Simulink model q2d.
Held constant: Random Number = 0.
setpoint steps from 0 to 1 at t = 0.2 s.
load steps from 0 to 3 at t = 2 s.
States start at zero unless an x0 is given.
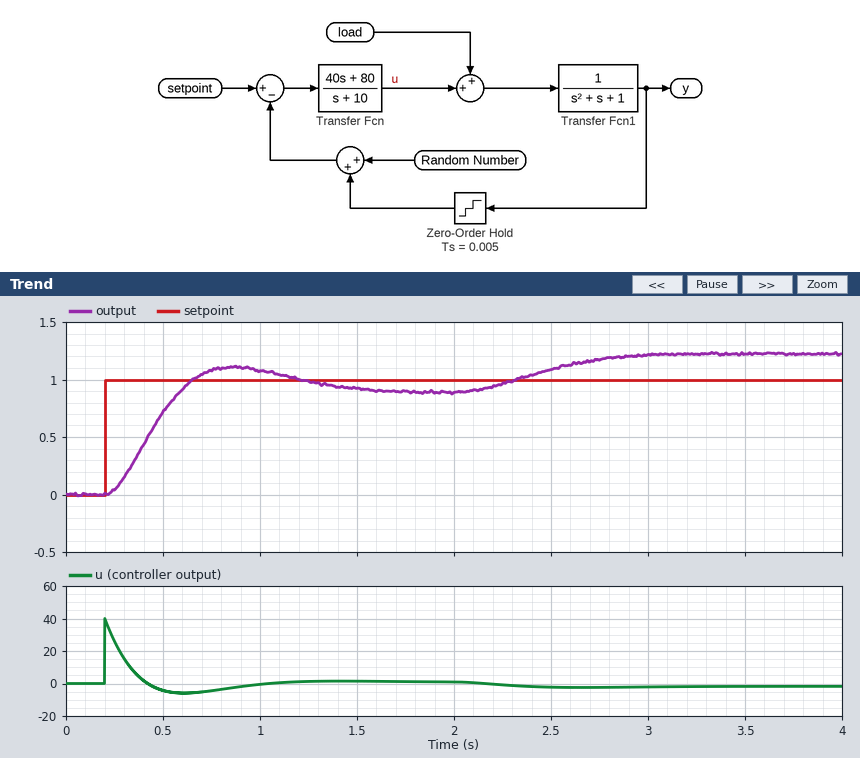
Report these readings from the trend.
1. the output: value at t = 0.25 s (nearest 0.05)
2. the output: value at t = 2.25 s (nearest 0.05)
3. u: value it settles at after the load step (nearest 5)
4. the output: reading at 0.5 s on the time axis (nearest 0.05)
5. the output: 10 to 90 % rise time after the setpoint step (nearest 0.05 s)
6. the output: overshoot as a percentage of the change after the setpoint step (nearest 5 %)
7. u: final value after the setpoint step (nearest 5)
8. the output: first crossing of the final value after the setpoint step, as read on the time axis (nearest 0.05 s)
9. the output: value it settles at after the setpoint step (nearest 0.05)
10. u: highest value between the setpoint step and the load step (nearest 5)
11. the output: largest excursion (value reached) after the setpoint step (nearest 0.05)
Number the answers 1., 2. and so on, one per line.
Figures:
1. 0.05
2. 0.95
3. 0
4. 0.70
5. 0.25 s
6. 25 %
7. 0
8. 0.60 s
9. 0.90
10. 40
11. 1.10
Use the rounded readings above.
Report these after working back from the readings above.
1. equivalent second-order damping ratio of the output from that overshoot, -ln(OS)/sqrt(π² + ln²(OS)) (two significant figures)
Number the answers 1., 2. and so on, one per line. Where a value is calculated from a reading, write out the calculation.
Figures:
1. ln(0.25) = -1.386; 1.386 / sqrt(9.870 + 1.922) = 0.40
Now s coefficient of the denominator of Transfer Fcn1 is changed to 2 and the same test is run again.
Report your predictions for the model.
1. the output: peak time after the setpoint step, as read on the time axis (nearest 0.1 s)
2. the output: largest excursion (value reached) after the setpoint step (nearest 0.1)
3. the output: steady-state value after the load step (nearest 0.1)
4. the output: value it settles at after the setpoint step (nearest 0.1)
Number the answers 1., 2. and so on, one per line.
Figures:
1. 0.9 s
2. 1.0
3. 1.2
4. 0.9
